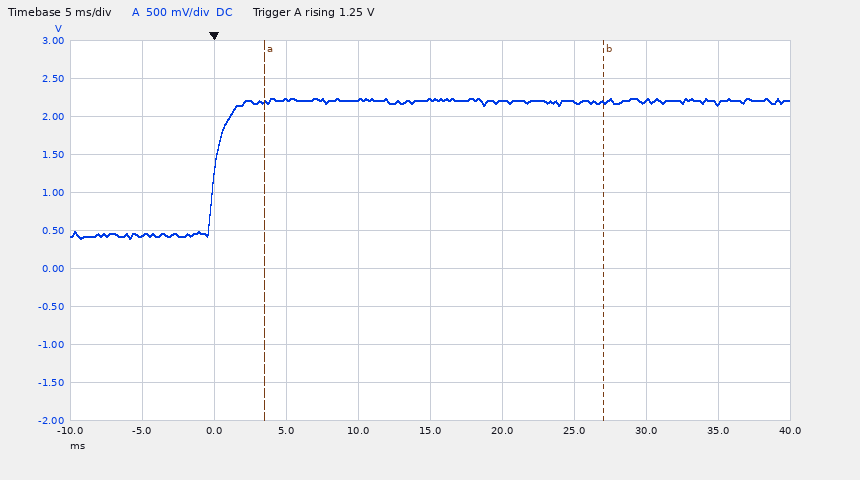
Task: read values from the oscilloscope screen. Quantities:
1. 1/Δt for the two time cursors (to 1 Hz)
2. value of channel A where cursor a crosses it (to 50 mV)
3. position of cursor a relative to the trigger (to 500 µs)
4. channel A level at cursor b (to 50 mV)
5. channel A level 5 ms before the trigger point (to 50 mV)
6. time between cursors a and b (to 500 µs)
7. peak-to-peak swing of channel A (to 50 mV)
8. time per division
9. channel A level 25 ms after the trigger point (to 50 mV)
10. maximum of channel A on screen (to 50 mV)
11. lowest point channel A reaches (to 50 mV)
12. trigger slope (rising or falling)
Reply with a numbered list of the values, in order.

1. 43 Hz
2. 2.20 V
3. +3.5 ms
4. 2.20 V
5. 450 mV
6. 23.5 ms
7. 1.85 V
8. 5 ms
9. 2.20 V
10. 2.25 V
11. 400 mV
12. rising
